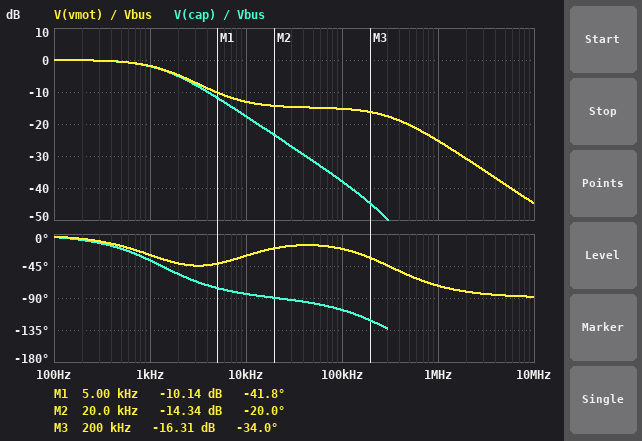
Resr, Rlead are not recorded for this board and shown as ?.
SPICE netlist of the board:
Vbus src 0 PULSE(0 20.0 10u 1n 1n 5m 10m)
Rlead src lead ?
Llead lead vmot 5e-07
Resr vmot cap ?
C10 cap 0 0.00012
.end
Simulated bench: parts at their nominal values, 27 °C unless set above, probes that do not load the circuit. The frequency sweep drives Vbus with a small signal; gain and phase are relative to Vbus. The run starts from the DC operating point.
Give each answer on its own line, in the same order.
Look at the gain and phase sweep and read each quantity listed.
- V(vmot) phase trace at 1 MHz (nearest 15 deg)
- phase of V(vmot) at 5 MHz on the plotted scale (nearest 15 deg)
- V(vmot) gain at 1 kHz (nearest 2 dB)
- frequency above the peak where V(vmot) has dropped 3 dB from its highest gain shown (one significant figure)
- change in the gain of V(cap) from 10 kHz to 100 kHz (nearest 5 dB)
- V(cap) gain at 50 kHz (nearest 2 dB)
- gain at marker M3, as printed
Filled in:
-75 deg
-90 deg
-2 dB
1 kHz
-20 dB
-32 dB
-16.31 dB
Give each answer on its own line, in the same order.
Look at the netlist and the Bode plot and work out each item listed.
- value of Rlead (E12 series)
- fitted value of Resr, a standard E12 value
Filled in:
0.82 Ω
0.18 Ω
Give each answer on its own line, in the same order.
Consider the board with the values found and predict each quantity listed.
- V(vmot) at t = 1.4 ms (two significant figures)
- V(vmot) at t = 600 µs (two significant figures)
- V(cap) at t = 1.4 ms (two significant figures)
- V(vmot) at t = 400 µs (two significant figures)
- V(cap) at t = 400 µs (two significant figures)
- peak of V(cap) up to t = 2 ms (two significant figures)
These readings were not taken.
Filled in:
20 V
20 V
20 V
19 V
19 V
20 V
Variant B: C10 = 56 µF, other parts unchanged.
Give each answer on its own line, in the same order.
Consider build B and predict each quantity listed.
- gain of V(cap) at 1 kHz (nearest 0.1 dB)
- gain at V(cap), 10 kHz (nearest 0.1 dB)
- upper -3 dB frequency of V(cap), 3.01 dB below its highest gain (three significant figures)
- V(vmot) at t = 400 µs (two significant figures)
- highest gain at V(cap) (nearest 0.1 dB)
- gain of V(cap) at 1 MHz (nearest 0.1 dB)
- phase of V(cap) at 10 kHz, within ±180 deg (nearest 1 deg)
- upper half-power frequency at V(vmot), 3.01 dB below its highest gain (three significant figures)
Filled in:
-0.5 dB
-11.2 dB
2.87 kHz
20 V
0 dB
-61.3 dB
-76 deg
2.97 kHz
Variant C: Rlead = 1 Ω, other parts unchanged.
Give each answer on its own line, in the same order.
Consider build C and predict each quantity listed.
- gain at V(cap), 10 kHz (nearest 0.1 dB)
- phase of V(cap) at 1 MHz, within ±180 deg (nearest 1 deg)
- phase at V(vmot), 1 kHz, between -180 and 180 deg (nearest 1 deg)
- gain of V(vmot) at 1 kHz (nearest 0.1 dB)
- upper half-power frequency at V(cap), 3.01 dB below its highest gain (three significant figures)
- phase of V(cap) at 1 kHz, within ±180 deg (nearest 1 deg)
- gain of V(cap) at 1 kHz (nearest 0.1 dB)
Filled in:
-19.0 dB
-159 deg
-34 deg
-2.4 dB
1.13 kHz
-42 deg
-2.5 dB
